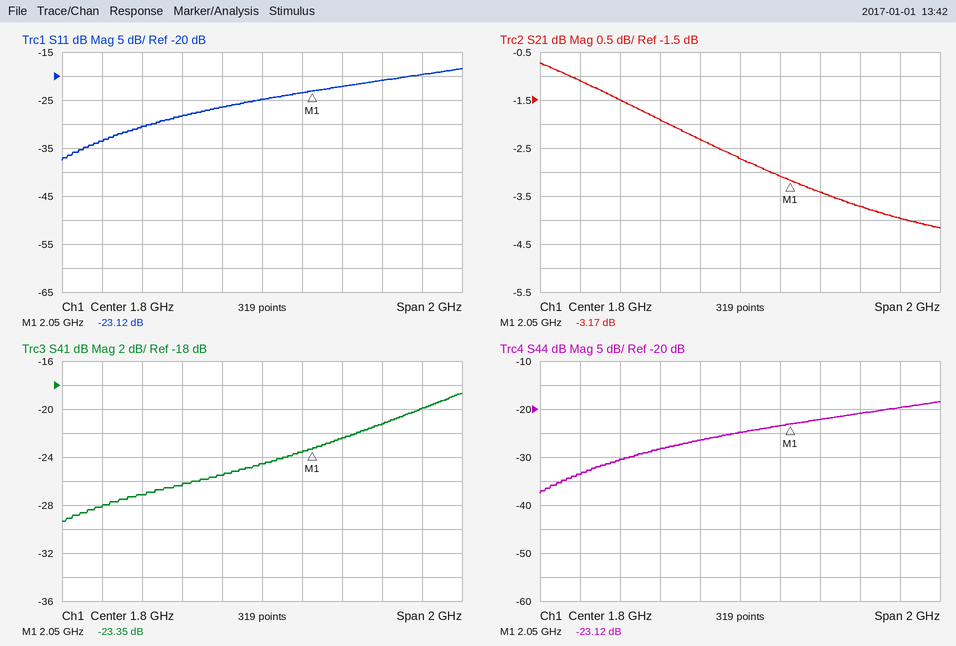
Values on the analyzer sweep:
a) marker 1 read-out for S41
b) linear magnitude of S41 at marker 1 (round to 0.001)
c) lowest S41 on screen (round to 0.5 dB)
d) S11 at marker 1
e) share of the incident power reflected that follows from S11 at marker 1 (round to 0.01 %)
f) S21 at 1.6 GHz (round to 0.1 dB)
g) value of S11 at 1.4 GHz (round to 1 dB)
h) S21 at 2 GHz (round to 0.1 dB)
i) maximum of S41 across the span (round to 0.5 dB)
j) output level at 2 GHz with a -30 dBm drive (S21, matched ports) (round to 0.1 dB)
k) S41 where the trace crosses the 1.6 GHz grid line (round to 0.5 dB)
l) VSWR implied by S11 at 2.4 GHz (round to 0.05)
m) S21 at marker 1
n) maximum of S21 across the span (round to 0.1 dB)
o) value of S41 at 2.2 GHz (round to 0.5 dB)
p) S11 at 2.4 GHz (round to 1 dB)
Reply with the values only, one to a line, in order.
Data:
-23.35 dB
0.068
-29.5 dB
-23.12 dB
0.49 %
-2.3 dB
-28 dB
-3.1 dB
-18.5 dB
-33.1 dBm
-25.5 dB
1.20
-3.17 dB
-0.7 dB
-22.5 dB
-21 dB
